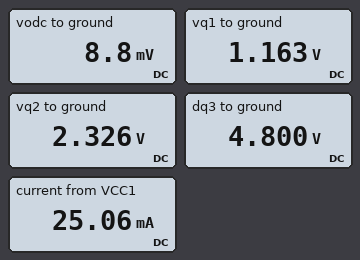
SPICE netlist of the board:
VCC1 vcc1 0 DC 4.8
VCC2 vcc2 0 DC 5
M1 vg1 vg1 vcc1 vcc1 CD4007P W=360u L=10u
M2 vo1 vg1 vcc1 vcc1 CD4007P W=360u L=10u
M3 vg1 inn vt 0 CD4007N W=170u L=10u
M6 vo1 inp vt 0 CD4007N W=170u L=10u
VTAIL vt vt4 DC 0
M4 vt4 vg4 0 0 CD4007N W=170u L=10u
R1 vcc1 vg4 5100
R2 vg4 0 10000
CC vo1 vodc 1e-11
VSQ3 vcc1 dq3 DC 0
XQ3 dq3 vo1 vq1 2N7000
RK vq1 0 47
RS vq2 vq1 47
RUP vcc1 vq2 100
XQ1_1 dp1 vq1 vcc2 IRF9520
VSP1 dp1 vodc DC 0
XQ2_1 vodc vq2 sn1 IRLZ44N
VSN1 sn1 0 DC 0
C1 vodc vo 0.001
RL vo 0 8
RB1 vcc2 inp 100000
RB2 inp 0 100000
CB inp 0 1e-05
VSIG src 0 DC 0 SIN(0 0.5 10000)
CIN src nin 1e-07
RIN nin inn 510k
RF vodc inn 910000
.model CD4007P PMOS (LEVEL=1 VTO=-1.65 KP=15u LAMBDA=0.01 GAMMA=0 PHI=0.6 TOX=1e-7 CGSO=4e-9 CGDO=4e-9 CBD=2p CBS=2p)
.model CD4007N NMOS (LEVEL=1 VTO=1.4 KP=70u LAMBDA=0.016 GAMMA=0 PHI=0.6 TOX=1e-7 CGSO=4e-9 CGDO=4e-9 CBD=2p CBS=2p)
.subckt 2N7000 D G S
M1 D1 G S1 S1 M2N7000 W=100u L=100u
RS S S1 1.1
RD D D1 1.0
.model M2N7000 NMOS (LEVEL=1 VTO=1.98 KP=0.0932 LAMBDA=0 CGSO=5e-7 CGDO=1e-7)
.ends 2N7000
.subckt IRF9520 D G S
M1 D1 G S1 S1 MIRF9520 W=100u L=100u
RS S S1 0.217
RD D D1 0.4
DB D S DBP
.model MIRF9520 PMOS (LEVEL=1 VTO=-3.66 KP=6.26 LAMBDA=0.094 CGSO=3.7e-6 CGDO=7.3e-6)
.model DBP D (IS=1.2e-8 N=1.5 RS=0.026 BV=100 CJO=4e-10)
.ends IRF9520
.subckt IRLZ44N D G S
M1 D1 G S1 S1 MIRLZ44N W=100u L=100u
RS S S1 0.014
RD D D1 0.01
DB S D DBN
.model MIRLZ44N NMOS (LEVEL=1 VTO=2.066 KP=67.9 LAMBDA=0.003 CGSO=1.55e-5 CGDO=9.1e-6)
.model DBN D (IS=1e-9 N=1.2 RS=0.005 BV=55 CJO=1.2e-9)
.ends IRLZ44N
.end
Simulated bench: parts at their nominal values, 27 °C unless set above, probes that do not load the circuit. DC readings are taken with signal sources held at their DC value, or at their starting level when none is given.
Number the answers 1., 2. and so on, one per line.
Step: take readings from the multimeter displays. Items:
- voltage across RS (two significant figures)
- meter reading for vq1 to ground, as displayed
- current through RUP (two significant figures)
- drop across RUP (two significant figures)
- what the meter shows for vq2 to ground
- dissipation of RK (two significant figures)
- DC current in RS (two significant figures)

1. 1.2 V
2. 1.163 V
3. 25 mA
4. 2.5 V
5. 2.326 V
6. 29 mW
7. 25 mA
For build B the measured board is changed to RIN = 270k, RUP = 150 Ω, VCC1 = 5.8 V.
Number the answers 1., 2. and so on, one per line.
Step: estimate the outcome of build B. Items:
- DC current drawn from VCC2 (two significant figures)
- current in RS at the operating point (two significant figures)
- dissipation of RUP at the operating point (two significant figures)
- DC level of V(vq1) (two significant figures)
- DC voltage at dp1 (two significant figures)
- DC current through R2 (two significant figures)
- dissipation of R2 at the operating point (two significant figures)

1. 160 mA
2. 24 mA
3. 85 mW
4. 1.1 V
5. 19 mV
6. 380 µA
7. 1.5 mW
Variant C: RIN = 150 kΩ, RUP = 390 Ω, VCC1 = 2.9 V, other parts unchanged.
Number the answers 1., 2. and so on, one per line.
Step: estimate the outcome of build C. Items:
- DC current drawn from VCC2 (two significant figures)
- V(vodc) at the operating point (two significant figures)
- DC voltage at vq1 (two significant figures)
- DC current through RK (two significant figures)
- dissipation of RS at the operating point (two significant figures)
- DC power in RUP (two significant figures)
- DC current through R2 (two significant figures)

1. 25 µA
2. 5.0 V
3. 280 mV
4. 6.0 mA
5. 1.7 mW
6. 14 mW
7. 190 µA
